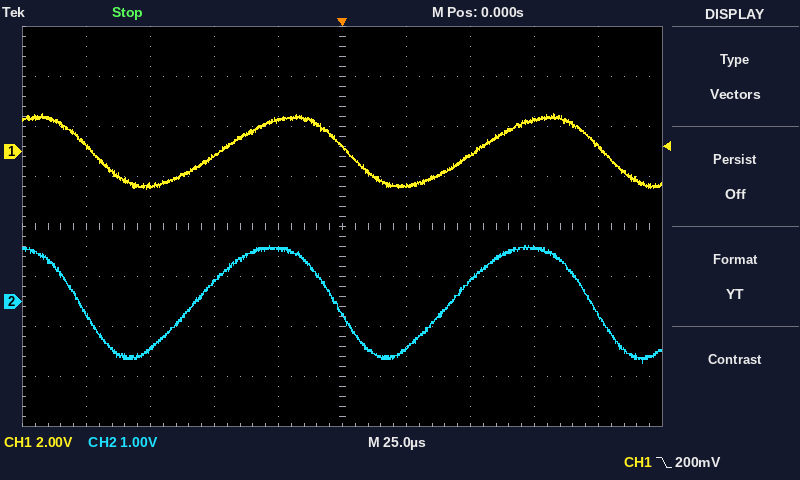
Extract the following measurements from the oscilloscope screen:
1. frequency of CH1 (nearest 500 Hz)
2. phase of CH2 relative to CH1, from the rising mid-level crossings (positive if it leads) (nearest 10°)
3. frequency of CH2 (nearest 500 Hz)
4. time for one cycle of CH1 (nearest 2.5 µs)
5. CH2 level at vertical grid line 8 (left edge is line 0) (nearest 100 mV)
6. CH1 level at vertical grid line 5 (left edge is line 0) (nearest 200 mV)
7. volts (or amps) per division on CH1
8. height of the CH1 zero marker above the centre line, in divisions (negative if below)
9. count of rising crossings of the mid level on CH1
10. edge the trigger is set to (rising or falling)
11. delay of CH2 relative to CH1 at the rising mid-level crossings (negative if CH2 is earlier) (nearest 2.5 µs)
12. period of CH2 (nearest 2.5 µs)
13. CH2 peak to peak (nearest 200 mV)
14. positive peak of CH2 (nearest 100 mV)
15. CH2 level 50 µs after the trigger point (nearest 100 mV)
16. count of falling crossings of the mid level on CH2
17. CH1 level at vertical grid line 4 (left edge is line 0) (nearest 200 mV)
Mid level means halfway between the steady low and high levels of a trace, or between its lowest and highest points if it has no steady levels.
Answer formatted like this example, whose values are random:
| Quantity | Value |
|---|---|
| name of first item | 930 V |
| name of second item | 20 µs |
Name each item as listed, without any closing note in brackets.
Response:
| Quantity | Value |
|---|---|
| frequency of CH1 | 10.0 kHz |
| phase of CH2 relative to CH1, from the rising mid-level crossings (positive if it leads) | +40° |
| frequency of CH2 | 10.0 kHz |
| time for one cycle of CH1 | 100.0 µs |
| CH2 level at vertical grid line 8 (left edge is line 0) | 1.1 V |
| CH1 level at vertical grid line 5 (left edge is line 0) | 200 mV |
| volts (or amps) per division on CH1 | 2 V |
| height of the CH1 zero marker above the centre line, in divisions | +1.5 div |
| count of rising crossings of the mid level on CH1 | 2 |
| edge the trigger is set to | falling |
| delay of CH2 relative to CH1 at the rising mid-level crossings (negative if CH2 is earlier) | -10.0 µs |
| period of CH2 | 100.0 µs |
| CH2 peak to peak | 2.4 V |
| positive peak of CH2 | 1.1 V |
| CH2 level 50 µs after the trigger point | 400 mV |
| count of falling crossings of the mid level on CH2 | 3 |
| CH1 level at vertical grid line 4 (left edge is line 0) | 1.2 V |
